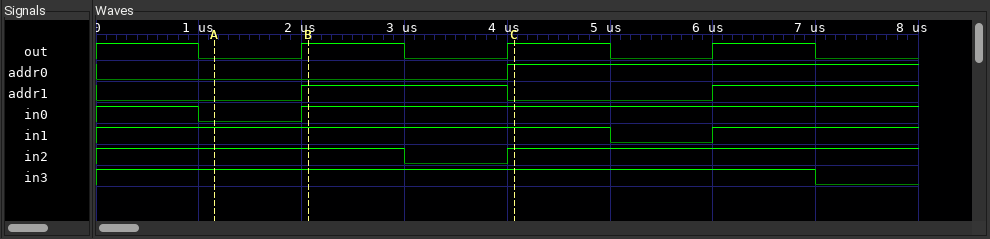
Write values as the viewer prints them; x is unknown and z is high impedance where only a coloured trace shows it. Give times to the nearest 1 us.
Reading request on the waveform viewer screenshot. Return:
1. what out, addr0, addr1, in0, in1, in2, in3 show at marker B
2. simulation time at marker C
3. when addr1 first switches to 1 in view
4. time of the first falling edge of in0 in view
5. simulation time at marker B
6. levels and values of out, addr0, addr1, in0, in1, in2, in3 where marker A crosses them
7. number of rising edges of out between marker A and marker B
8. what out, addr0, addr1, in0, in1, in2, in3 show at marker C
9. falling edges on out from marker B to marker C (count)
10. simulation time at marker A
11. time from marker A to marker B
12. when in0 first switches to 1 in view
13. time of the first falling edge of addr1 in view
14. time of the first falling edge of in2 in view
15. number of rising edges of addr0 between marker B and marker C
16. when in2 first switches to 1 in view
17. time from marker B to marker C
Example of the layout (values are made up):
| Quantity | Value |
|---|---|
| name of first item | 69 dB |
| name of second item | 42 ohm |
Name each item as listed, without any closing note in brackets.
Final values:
| Quantity | Value |
|---|---|
| what out, addr0, addr1, in0, in1, in2, in3 show at marker B | out=1, addr0=0, addr1=1, in0=1, in1=1, in2=1, in3=1 |
| simulation time at marker C | 4 us |
| when addr1 first switches to 1 in view | 2 us |
| time of the first falling edge of in0 in view | 1 us |
| simulation time at marker B | 2 us |
| levels and values of out, addr0, addr1, in0, in1, in2, in3 where marker A crosses them | out=0, addr0=0, addr1=0, in0=0, in1=1, in2=1, in3=1 |
| number of rising edges of out between marker A and marker B | 1 |
| what out, addr0, addr1, in0, in1, in2, in3 show at marker C | out=1, addr0=1, addr1=0, in0=1, in1=1, in2=1, in3=1 |
| falling edges on out from marker B to marker C | 1 |
| simulation time at marker A | 1 us |
| time from marker A to marker B | 1 us |
| when in0 first switches to 1 in view | 2 us |
| time of the first falling edge of addr1 in view | 4 us |
| time of the first falling edge of in2 in view | 3 us |
| number of rising edges of addr0 between marker B and marker C | 1 |
| when in2 first switches to 1 in view | 4 us |
| time from marker B to marker C | 2 us |
